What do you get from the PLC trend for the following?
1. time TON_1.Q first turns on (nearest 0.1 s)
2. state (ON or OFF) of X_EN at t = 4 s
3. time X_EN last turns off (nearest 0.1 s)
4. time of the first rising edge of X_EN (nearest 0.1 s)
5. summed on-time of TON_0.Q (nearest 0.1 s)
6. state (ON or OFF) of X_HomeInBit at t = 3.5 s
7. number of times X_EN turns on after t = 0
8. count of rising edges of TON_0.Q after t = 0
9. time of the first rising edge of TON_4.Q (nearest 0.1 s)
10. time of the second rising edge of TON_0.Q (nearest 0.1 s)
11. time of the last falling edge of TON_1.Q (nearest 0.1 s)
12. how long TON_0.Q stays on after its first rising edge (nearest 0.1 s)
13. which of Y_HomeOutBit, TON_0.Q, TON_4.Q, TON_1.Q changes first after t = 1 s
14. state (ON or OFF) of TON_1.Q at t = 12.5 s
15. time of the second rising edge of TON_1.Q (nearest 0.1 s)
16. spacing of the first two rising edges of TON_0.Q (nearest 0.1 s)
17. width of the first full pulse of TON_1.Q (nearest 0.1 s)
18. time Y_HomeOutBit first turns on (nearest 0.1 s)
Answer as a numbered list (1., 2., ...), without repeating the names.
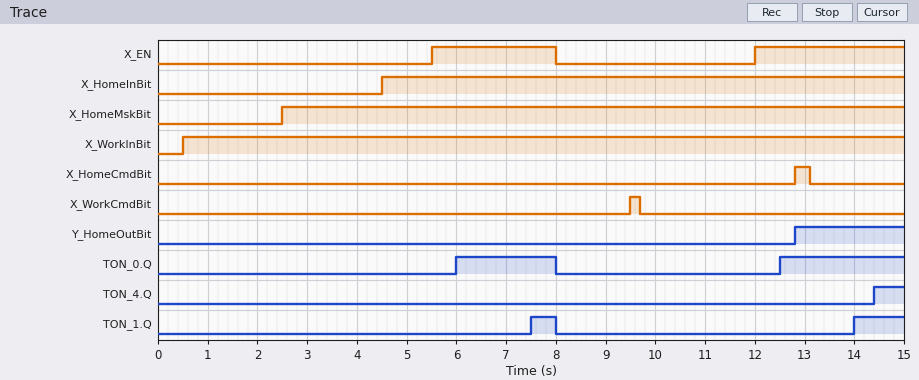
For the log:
1. 7.5 s
2. OFF
3. 8.0 s
4. 5.5 s
5. 4.5 s
6. OFF
7. 2
8. 2
9. 14.4 s
10. 12.5 s
11. 8.0 s
12. 2.0 s
13. TON_0.Q
14. OFF
15. 14.0 s
16. 6.5 s
17. 0.5 s
18. 12.8 s
